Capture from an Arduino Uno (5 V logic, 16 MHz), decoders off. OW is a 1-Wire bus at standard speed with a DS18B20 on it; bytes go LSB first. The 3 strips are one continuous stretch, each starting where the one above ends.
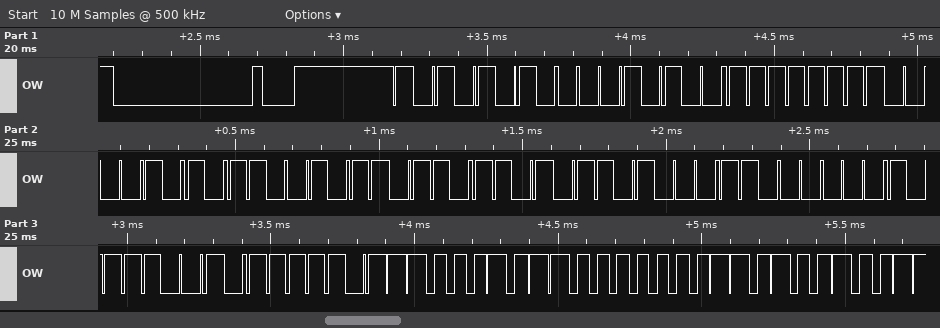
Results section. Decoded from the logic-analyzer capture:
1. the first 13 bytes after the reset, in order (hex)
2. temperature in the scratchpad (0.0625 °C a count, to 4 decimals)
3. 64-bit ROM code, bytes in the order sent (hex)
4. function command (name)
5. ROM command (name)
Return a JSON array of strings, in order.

["55 28 FF 50 D3 B6 16 03 9D BE A3 01 4B", "26.1875 °C", "28 FF 50 D3 B6 16 03 9D", "Read Scratchpad", "Match ROM"]
